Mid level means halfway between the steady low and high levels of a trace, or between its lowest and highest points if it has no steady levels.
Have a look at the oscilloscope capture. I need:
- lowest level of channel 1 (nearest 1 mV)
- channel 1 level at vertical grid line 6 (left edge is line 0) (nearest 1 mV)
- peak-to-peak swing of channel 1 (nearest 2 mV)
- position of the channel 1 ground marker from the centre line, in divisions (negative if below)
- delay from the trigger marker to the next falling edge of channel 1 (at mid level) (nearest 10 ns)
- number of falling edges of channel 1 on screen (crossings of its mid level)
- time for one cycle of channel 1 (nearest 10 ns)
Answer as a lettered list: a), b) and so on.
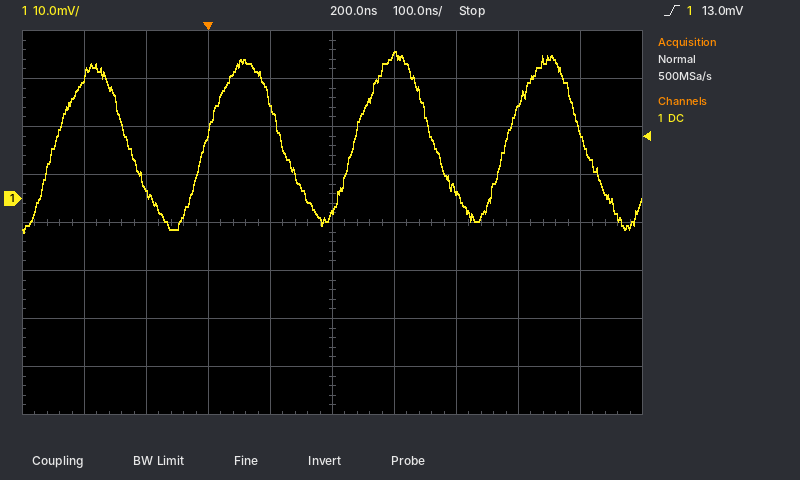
a) -7 mV
b) 30 mV
c) 38 mV
d) +0.5 div
e) 120 ns
f) 4
g) 240 ns
